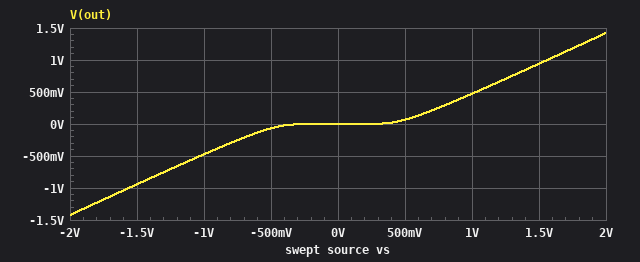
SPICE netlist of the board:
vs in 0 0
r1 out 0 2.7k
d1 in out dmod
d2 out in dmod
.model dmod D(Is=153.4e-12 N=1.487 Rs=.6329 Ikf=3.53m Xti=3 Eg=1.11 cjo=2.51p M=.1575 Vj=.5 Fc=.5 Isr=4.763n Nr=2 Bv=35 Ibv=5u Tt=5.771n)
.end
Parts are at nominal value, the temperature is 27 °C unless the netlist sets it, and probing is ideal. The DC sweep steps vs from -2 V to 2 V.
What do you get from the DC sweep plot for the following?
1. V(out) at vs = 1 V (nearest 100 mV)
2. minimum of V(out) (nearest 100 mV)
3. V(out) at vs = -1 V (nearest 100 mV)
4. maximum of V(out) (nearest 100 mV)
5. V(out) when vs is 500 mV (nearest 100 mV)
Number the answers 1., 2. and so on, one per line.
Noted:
1. 500 mV
2. -1.4 V
3. -500 mV
4. 1.4 V
5. 100 mV
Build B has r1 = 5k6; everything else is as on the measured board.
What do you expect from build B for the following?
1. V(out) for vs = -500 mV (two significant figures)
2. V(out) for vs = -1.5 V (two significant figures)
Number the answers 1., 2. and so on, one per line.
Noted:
1. -89 mV
2. -970 mV
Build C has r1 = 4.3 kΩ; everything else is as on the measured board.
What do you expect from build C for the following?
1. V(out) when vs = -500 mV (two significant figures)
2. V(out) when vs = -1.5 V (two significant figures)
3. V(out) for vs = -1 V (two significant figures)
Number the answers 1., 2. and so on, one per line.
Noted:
1. -81 mV
2. -960 mV
3. -490 mV
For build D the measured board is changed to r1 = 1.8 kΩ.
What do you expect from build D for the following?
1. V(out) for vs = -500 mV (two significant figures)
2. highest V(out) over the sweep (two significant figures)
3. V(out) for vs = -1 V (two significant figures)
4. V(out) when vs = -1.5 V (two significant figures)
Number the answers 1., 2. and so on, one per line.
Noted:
1. -56 mV
2. 1.4 V
3. -460 mV
4. -920 mV
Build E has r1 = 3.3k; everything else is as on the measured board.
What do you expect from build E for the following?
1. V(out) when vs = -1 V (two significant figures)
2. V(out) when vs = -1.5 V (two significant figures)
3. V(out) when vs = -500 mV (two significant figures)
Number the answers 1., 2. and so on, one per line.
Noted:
1. -480 mV
2. -950 mV
3. -73 mV
